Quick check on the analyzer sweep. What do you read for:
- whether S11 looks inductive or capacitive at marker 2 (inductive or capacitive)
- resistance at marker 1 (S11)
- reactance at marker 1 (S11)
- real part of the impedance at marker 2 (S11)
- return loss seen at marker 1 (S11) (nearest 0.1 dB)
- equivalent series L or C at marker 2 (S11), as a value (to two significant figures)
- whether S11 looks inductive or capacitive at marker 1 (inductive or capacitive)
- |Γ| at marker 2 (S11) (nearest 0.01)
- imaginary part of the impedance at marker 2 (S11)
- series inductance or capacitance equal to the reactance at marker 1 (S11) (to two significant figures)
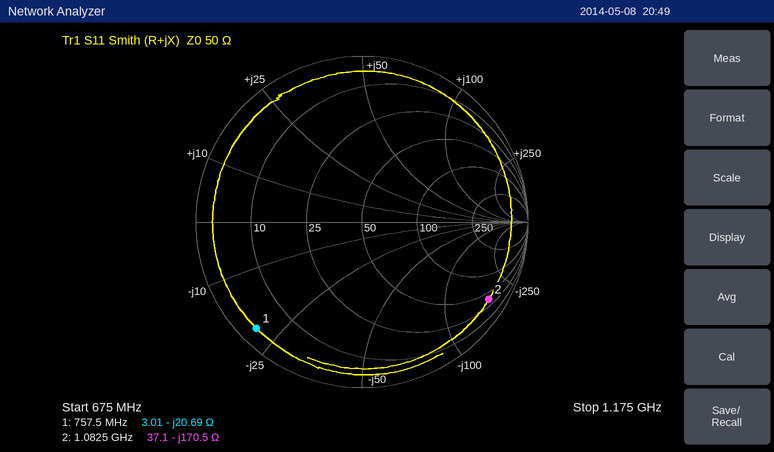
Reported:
capacitive
3.01 Ω
-20.69 Ω
37.1 Ω
0.9 dB
860 fF
capacitive
0.89
-170.5 Ω
10 pF
